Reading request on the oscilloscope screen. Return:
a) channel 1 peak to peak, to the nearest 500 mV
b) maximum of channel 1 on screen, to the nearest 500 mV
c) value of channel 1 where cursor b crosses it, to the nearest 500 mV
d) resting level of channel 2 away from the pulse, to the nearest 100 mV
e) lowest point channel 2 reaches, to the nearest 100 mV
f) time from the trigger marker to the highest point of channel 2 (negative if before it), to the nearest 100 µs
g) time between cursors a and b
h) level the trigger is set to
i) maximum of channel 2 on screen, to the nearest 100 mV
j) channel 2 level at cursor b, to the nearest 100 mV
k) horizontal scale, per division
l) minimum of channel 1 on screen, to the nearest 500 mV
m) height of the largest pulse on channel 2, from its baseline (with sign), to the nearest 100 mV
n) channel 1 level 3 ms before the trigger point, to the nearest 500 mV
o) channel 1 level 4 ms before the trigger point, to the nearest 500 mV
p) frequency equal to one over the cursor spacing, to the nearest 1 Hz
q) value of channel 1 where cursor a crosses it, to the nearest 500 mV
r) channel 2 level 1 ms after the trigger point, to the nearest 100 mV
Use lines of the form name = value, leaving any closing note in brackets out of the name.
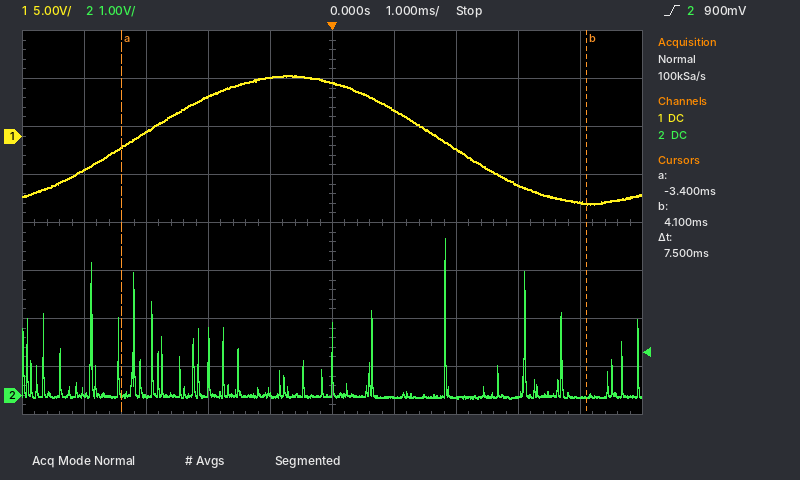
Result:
channel 1 peak to peak, to the nearest 500 mV = 13.5 V
maximum of channel 1 on screen, to the nearest 500 mV = 6.5 V
value of channel 1 where cursor b crosses it, to the nearest 500 mV = -7.0 V
resting level of channel 2 away from the pulse, to the nearest 100 mV = 0.0 V
lowest point channel 2 reaches, to the nearest 100 mV = -100 mV
time from the trigger marker to the highest point of channel 2 (negative if before it), to the nearest 100 µs = +1.8 ms
time between cursors a and b = 7.5 ms
level the trigger is set to = 900 mV
maximum of channel 2 on screen, to the nearest 100 mV = 3.3 V
channel 2 level at cursor b, to the nearest 100 mV = 0.0 V
horizontal scale, per division = 1 ms
minimum of channel 1 on screen, to the nearest 500 mV = -7.0 V
height of the largest pulse on channel 2, from its baseline (with sign), to the nearest 100 mV = +3.3 V
channel 1 level 3 ms before the trigger point, to the nearest 500 mV = 500 mV
channel 1 level 4 ms before the trigger point, to the nearest 500 mV = -3.5 V
frequency equal to one over the cursor spacing, to the nearest 1 Hz = 133 Hz
value of channel 1 where cursor a crosses it, to the nearest 500 mV = -1.0 V
channel 2 level 1 ms after the trigger point, to the nearest 100 mV = 0.0 V
